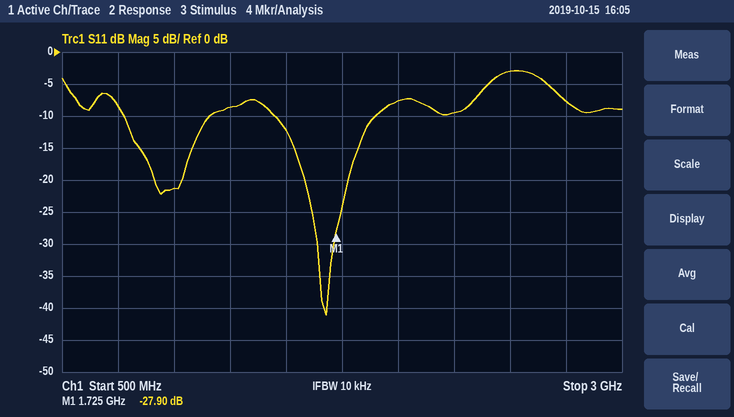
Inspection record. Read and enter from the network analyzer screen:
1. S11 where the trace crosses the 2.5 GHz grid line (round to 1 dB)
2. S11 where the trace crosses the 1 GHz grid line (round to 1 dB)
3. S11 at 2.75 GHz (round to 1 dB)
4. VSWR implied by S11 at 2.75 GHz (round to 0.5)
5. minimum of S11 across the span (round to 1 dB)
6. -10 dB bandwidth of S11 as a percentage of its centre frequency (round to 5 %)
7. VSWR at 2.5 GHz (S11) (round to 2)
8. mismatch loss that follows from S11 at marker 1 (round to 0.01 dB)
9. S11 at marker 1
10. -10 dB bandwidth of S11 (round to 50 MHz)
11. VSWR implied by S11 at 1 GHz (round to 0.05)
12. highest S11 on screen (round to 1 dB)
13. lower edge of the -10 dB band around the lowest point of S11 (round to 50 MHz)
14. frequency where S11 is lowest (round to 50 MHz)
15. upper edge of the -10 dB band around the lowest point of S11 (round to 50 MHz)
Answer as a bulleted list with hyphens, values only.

- -3 dB
- -21 dB
- -8 dB
- 2.5
- -41 dB
- 25 %
- 6
- 0.01 dB
- -27.90 dB
- 450 MHz
- 1.20
- -3 dB
- 1.45 GHz
- 1.70 GHz
- 1.90 GHz
